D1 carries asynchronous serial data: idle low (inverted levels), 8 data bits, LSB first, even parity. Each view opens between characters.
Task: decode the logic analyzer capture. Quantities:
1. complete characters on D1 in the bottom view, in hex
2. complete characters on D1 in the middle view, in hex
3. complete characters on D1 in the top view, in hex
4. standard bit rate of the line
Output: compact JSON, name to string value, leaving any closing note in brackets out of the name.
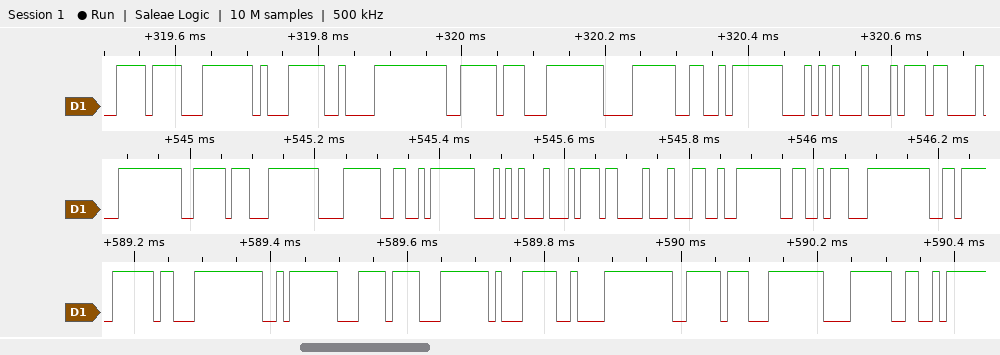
{"complete characters on D1 in the bottom view, in hex": "20, 00, 01, 08, 40, B0, 00, 10, 80, 60", "complete characters on D1 in the middle view, in hex": "00, 10, 80, 60, 01, 75, 91, 77, 03, 16, 00", "complete characters on D1 in the top view, in hex": "08, 40, B0, 00, 10, 80, 60, 01, 75, 91", "standard bit rate of the line": "100000 baud"}
